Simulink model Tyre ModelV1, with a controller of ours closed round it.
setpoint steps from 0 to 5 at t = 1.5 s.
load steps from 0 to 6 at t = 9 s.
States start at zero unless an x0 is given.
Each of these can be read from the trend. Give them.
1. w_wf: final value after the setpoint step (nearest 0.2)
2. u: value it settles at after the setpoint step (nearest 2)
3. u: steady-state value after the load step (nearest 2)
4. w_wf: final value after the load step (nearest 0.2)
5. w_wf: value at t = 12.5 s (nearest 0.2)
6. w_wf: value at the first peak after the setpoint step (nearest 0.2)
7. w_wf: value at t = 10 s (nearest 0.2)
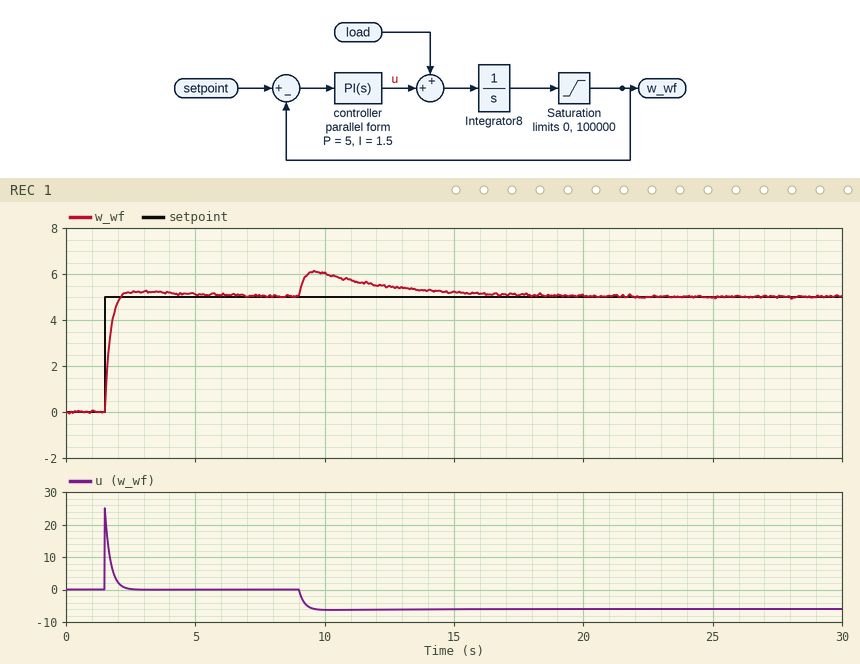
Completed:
5.0
0
-6
5.0
5.4
5.2
6.0
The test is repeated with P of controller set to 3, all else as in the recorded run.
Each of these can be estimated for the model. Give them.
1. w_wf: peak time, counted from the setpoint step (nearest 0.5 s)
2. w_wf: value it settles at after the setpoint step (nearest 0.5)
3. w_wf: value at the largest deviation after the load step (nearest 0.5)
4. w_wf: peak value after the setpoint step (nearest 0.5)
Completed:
1.5 s
5.0
6.5
5.5
